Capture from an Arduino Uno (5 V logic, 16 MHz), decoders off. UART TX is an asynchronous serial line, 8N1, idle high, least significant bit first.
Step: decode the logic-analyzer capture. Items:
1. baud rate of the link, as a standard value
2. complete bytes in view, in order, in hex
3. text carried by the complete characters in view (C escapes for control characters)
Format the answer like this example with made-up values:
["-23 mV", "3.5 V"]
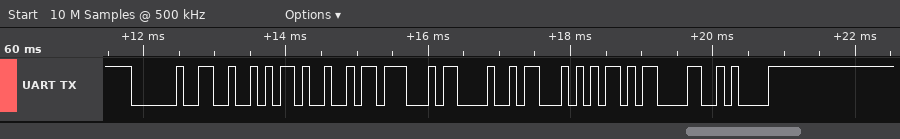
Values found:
["9600 baud", "0x20 0x52 0x49 0x47 0x48 0x54 0x0D 0x0A", "\" RIGHT\\r\\n\""]
